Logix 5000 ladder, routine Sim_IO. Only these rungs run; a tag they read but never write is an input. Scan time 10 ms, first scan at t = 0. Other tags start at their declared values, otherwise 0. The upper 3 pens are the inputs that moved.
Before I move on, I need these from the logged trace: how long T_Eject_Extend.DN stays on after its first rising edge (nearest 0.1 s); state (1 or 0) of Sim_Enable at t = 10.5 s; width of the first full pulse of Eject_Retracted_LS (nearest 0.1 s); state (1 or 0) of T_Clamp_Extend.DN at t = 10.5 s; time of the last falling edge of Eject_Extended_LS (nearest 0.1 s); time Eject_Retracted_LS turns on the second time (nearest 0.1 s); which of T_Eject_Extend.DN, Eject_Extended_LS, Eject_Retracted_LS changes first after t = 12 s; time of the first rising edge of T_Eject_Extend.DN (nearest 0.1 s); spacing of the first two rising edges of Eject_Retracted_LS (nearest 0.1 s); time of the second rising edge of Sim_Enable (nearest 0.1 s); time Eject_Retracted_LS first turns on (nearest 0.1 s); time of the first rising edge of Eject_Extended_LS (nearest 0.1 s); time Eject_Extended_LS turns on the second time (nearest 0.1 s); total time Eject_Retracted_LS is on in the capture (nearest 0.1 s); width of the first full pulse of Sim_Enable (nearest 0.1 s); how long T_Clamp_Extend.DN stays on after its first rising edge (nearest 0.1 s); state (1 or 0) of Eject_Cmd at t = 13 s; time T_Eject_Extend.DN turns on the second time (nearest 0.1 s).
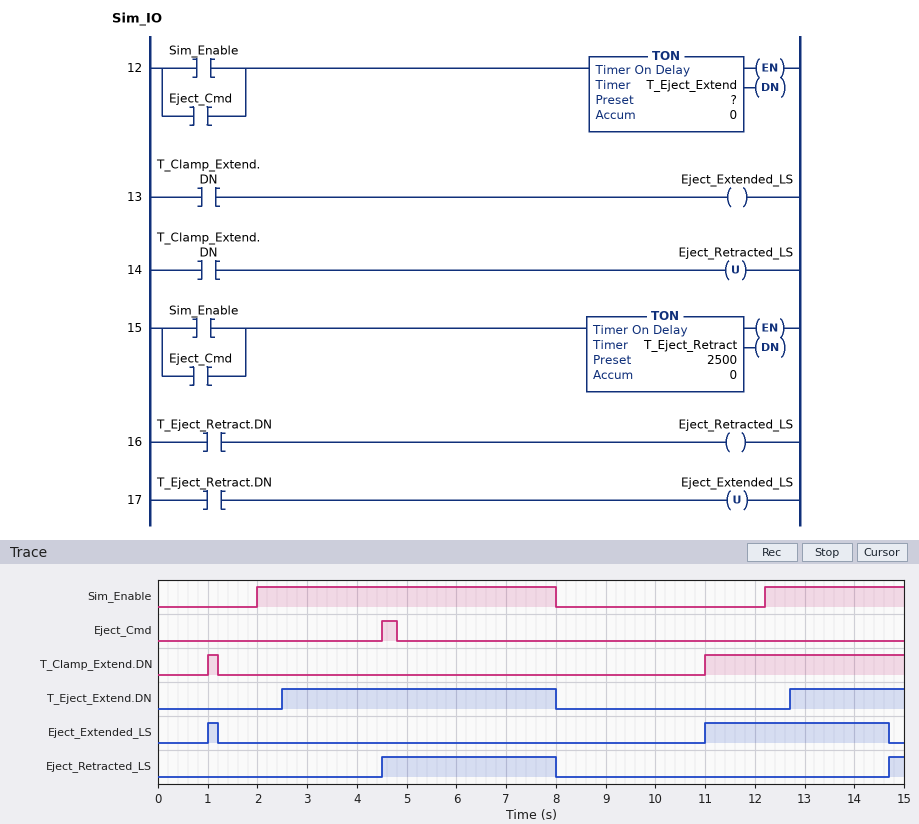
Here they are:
5.5 s
0
3.5 s
0
14.7 s
14.7 s
T_Eject_Extend.DN
2.5 s
10.2 s
12.2 s
4.5 s
1.0 s
11.0 s
3.8 s
6.0 s
0.2 s
0
12.7 s
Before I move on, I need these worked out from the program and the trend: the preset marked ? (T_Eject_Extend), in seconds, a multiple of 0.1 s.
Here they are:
0.5 s
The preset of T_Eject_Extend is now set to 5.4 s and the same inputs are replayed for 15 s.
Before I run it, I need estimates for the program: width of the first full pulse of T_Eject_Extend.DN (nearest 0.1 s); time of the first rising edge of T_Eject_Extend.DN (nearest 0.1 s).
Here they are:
0.6 s
7.4 s
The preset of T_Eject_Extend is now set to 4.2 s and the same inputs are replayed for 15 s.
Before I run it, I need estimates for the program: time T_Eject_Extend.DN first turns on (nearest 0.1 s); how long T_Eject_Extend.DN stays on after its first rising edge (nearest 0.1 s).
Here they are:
6.2 s
1.8 s
